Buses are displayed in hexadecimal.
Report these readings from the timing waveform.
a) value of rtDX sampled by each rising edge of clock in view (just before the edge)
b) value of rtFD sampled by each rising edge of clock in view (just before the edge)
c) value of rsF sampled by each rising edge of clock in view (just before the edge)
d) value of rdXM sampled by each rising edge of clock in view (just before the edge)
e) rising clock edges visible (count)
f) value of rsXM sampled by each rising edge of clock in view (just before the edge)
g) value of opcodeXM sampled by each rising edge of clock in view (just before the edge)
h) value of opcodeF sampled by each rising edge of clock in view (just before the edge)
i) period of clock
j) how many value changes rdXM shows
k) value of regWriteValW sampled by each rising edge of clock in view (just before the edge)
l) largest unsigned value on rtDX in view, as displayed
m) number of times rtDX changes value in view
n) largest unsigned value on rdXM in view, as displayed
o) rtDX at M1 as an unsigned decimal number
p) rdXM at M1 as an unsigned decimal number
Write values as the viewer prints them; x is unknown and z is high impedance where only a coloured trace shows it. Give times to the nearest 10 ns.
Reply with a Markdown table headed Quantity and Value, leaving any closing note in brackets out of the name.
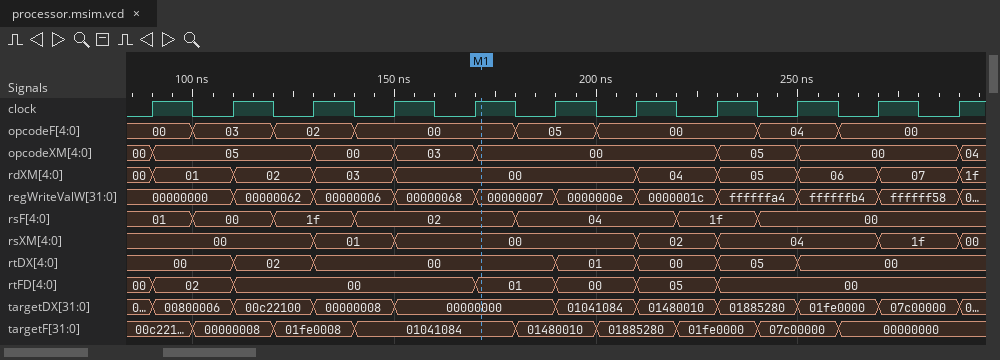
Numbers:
| Quantity | Value |
|---|---|
| value of rtDX sampled by each rising edge of clock in view | 00, 00, 02, 00, 00, 00, 01, 00, 05, 00, 00 |
| value of rtFD sampled by each rising edge of clock in view | 00, 02, 00, 00, 00, 01, 00, 05, 00, 00, 00 |
| value of rsF sampled by each rising edge of clock in view | 01, 00, 1f, 02, 02, 04, 04, 1f, 00, 00, 00 |
| value of rdXM sampled by each rising edge of clock in view | 00, 01, 02, 03, 00, 00, 00, 04, 05, 06, 07 |
| rising clock edges visible | 11 |
| value of rsXM sampled by each rising edge of clock in view | 00, 00, 00, 01, 00, 00, 00, 02, 04, 04, 1f |
| value of opcodeXM sampled by each rising edge of clock in view | 00, 05, 05, 00, 03, 00, 00, 00, 05, 00, 00 |
| value of opcodeF sampled by each rising edge of clock in view | 00, 03, 02, 00, 00, 05, 00, 00, 04, 00, 00 |
| period of clock | 20 ns |
| how many value changes rdXM shows | 9 |
| value of regWriteValW sampled by each rising edge of clock in view | 00000000, 00000000, 00000062, 00000006, 00000068, 00000007, 0000000e, 0000001c, ffffffa4, ffffffb4, ffffff58 |
| largest unsigned value on rtDX in view, as displayed | 05 |
| number of times rtDX changes value in view | 6 |
| largest unsigned value on rdXM in view, as displayed | 1f |
| rtDX at M1 as an unsigned decimal number | 0 |
| rdXM at M1 as an unsigned decimal number | 0 |
